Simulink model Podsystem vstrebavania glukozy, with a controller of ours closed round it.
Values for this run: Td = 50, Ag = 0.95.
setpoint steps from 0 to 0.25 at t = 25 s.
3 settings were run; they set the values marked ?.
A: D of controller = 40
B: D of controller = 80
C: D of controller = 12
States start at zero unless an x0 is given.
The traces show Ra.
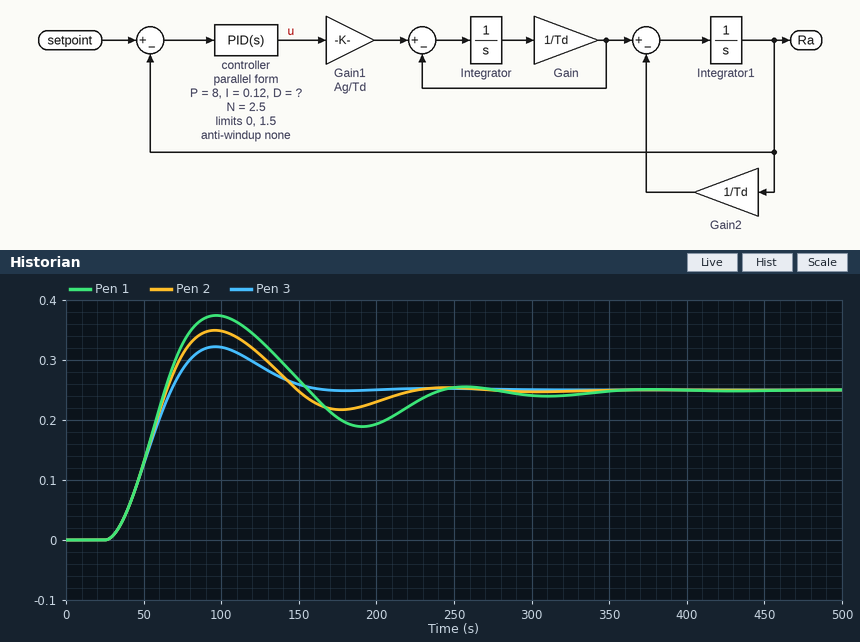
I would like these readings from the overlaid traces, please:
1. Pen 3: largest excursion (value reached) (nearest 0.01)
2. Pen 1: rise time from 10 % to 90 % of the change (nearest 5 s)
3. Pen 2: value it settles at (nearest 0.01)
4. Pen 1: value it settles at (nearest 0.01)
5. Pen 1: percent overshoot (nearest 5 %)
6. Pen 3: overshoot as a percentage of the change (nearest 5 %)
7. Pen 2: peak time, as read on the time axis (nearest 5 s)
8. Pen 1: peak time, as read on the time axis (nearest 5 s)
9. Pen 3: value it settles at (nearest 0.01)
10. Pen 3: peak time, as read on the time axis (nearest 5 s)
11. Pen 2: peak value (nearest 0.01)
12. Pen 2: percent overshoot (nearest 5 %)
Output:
0.32
25 s
0.25
0.25
50 %
30 %
95 s
95 s
0.25
95 s
0.35
40 %
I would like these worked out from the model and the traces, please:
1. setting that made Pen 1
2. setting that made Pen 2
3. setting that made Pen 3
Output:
C
A
B
